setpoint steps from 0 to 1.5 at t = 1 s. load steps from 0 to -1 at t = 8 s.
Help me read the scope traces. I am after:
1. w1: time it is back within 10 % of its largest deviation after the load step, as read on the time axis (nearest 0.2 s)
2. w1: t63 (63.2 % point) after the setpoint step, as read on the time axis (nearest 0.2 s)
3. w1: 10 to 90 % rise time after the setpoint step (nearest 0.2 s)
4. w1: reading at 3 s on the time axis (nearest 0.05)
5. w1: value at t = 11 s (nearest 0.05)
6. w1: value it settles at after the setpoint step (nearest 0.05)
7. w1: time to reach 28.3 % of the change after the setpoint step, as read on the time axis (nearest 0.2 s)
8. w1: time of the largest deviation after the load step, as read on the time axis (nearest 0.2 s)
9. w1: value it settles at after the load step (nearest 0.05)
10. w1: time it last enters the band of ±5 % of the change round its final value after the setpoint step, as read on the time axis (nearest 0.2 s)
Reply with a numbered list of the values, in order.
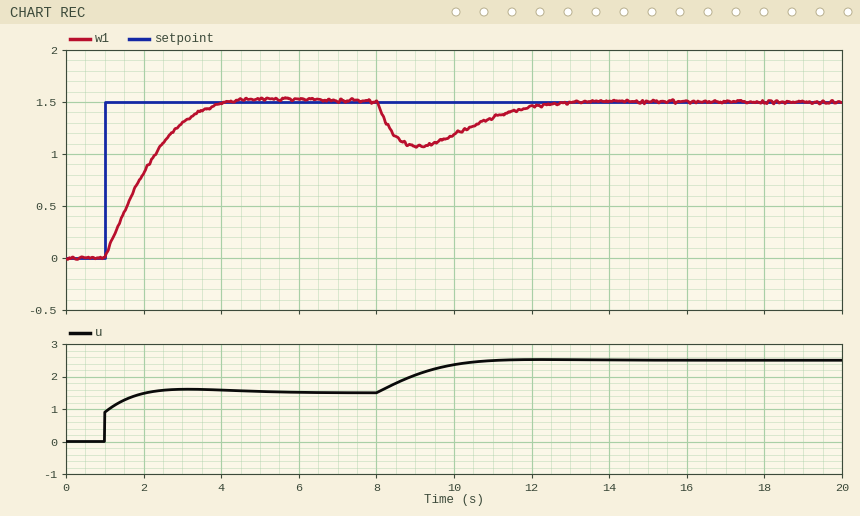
1. 12.0 s
2. 2.2 s
3. 2.0 s
4. 1.30
5. 1.35
6. 1.50
7. 1.4 s
8. 9.0 s
9. 1.50
10. 3.6 s
